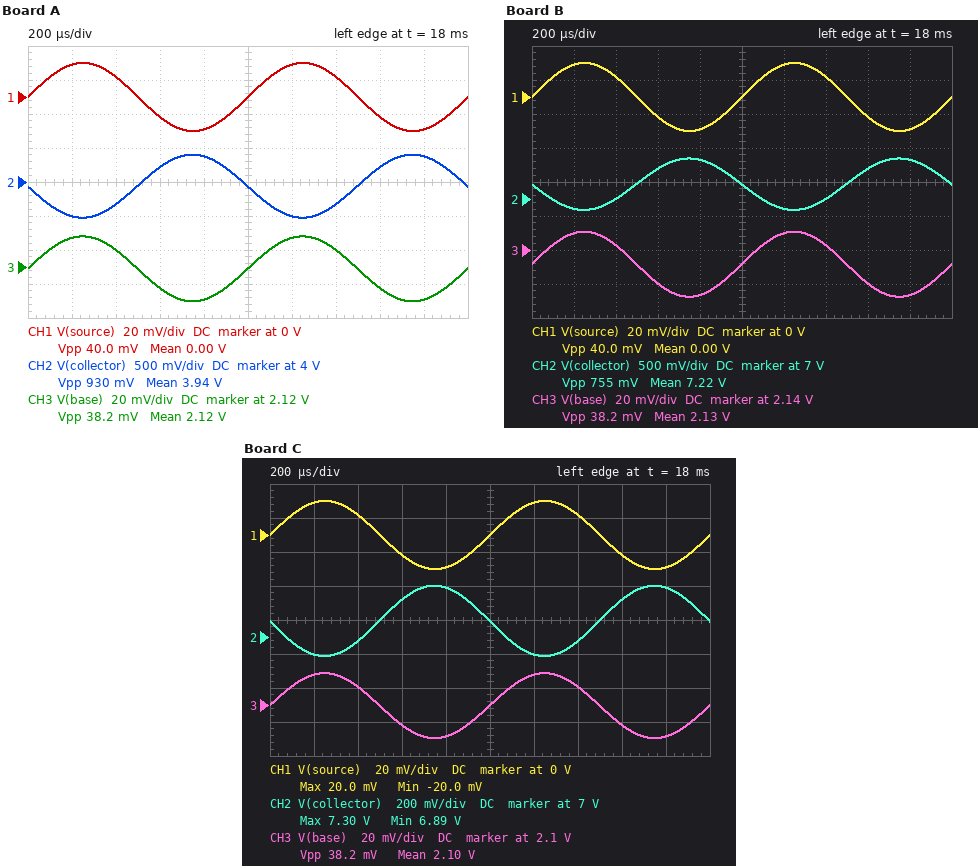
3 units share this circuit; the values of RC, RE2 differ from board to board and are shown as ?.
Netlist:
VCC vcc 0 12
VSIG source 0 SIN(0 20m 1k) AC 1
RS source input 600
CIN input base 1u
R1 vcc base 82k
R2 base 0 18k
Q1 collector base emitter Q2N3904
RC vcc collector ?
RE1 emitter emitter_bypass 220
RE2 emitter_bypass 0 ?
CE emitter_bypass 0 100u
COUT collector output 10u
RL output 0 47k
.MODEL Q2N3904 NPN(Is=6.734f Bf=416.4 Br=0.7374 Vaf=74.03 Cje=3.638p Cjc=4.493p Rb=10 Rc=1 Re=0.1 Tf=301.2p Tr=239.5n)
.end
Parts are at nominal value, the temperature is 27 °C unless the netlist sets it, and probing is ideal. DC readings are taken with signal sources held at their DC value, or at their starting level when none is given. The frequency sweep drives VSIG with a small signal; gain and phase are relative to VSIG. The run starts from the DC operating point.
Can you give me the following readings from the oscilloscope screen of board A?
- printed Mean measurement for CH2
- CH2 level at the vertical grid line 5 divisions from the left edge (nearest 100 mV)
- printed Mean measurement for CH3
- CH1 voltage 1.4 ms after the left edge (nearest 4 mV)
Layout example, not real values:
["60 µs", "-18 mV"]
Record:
["3.94 V", "3.9 V", "2.12 V", "12 mV"]
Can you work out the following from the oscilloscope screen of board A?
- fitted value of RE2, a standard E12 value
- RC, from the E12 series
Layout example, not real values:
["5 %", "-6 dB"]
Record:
["1 kΩ", "6.8 kΩ"]
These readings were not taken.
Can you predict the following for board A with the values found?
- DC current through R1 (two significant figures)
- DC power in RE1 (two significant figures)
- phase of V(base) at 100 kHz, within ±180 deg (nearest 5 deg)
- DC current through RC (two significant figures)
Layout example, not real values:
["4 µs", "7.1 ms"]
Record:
["120 µA", "310 µW", "0 deg", "1.2 mA"]
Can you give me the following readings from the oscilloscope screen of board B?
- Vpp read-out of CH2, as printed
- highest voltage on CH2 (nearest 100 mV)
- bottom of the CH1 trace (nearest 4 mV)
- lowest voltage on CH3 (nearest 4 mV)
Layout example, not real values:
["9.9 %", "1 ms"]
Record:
["755 mV", "7.6 V", "-20 mV", "2.112 V"]
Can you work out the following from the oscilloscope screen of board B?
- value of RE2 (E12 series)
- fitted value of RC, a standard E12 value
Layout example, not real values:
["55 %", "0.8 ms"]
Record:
["1.5 kΩ", "5.6 kΩ"]
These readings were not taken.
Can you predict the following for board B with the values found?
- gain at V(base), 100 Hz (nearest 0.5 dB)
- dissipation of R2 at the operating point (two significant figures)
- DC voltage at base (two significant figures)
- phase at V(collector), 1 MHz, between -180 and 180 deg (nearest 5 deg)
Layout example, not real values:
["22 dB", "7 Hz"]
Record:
["-0.5 dB", "250 µW", "2.1 V", "165 deg"]
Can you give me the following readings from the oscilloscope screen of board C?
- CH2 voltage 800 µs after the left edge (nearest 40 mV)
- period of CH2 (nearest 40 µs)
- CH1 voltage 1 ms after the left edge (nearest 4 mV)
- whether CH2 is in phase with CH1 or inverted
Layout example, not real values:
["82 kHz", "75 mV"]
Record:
["7.28 V", "1.00 ms", "0 V", "inverted"]
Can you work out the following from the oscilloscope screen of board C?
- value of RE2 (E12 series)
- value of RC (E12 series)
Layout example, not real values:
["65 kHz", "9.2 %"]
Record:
["560 Ω", "2.7 kΩ"]
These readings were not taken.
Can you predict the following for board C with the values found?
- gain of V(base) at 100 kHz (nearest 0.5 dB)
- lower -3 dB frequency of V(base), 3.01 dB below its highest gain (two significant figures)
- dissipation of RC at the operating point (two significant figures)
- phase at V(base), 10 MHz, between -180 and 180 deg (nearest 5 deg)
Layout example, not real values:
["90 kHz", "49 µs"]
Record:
["-0.5 dB", "12 Hz", "8.9 mW", "-35 deg"]
